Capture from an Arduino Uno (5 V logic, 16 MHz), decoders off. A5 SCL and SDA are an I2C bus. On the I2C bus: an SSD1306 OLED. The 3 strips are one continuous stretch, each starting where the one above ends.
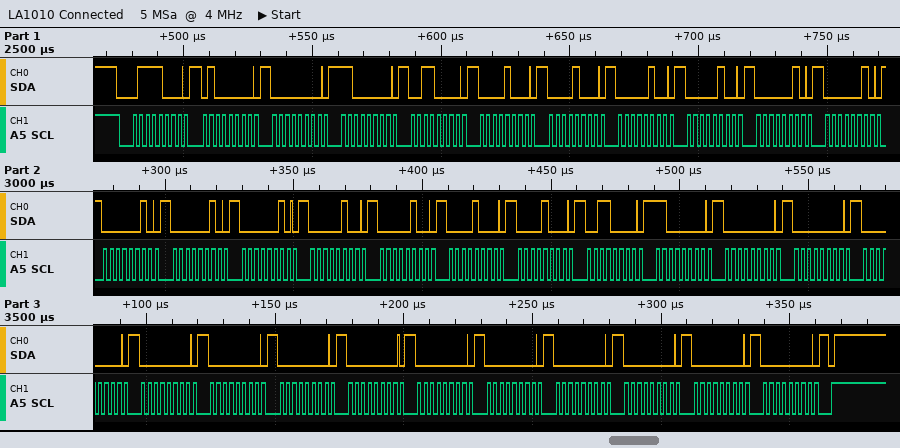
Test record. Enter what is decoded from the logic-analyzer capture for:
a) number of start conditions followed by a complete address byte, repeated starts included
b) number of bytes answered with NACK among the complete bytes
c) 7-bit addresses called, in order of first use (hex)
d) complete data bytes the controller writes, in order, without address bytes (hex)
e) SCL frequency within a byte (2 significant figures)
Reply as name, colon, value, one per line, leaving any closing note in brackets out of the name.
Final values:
number of start conditions followed by a complete address byte, repeated starts included: 1
number of bytes answered with NACK among the complete bytes: 0
7-bit addresses called, in order of first use: 0x3C
complete data bytes the controller writes, in order, without address bytes: 40 00 C0 30 08 08 04 04 02 02 02 02 02 04 04 08 08 30 C0 00 00 00 00 00 00 00 00 00 00 00 00 00
SCL frequency within a byte: 400 kHz
